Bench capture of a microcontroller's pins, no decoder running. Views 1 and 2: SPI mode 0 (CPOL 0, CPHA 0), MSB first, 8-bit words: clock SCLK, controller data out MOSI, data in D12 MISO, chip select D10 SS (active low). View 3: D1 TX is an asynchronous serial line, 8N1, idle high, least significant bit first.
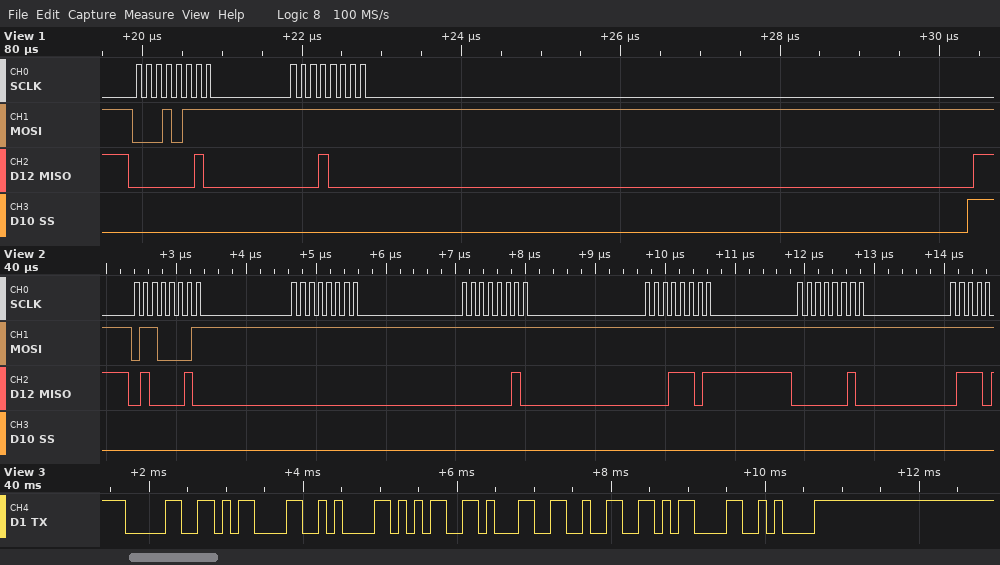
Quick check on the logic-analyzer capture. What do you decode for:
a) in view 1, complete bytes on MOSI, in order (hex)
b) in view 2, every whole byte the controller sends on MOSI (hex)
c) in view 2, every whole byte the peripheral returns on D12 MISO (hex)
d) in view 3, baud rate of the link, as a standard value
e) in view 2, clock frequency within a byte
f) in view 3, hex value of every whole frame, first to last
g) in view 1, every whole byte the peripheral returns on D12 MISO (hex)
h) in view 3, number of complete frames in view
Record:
17 FF
0x61 0xFF 0xFF 0xFF 0xFF
0x42 0x00 0x02 0x1D 0x02
9600 baud
8 MHz
30 0D 0A 35 31 32 0D 0A
02 10
8
